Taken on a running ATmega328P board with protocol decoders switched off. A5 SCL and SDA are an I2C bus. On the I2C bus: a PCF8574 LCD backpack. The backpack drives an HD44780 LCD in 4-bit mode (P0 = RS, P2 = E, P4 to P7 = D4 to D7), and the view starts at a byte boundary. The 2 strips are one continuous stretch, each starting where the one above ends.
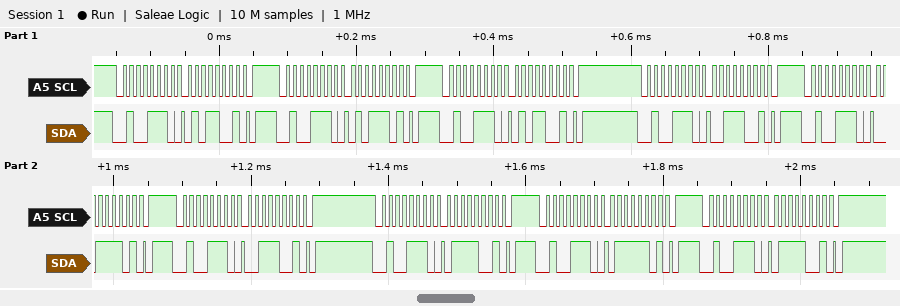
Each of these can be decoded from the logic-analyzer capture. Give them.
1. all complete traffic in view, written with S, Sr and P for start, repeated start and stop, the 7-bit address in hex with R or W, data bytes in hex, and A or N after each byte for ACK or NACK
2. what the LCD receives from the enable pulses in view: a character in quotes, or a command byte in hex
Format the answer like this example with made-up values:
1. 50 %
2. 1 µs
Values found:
1. S 27W A 59 A P S 27W A 5D A P S 27W A 59 A P S 27W A 39 A P S 27W A 3D A P S 27W A 39 A P S 27W A 79 A P S 27W A 7D A P S 27W A 79 A P
2. 'S'
